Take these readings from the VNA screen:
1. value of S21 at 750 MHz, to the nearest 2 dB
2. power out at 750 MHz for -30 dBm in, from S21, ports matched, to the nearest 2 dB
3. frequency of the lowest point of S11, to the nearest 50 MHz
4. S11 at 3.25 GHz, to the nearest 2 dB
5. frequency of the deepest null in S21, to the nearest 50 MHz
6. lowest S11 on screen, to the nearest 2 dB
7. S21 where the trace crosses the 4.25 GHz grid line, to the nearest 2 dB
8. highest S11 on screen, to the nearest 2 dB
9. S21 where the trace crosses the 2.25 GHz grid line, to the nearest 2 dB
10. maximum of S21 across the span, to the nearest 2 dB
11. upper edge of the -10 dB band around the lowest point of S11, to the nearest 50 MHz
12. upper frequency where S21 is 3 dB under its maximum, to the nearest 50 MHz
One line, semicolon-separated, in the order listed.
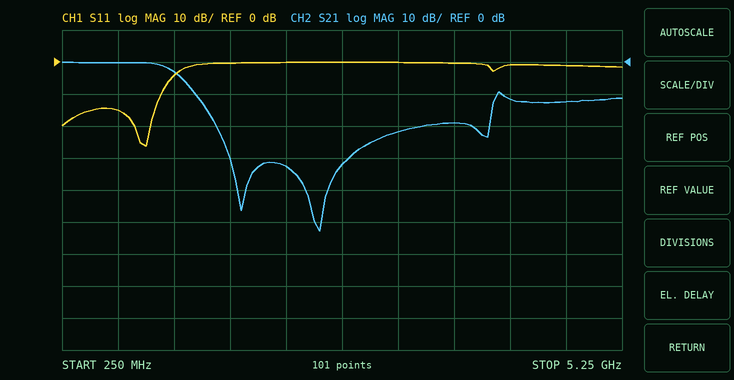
0 dB; -30 dBm; 1.00 GHz; 0 dB; 2.55 GHz; -26 dB; -12 dB; 0 dB; -32 dB; 0 dB; 1.15 GHz; 1.25 GHz
